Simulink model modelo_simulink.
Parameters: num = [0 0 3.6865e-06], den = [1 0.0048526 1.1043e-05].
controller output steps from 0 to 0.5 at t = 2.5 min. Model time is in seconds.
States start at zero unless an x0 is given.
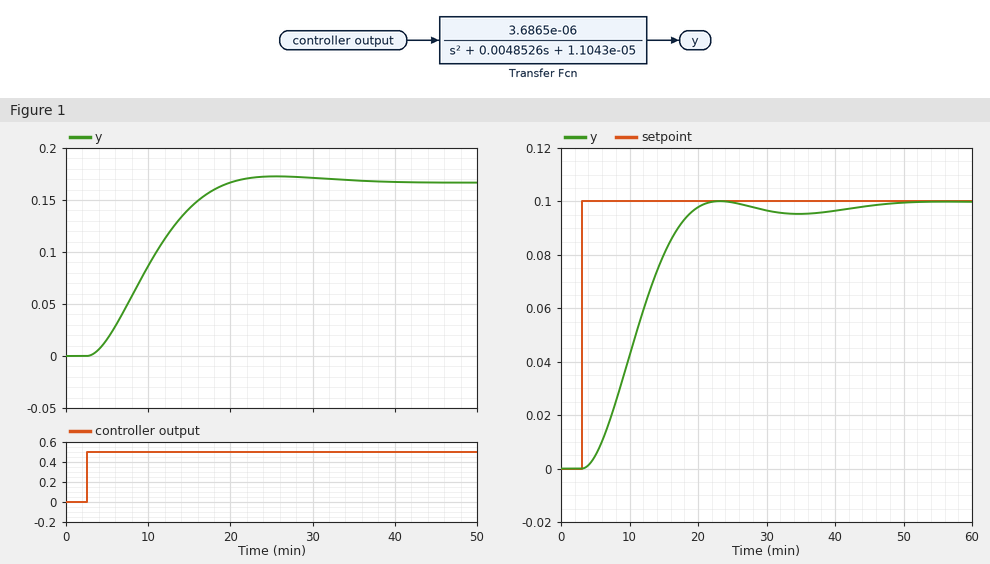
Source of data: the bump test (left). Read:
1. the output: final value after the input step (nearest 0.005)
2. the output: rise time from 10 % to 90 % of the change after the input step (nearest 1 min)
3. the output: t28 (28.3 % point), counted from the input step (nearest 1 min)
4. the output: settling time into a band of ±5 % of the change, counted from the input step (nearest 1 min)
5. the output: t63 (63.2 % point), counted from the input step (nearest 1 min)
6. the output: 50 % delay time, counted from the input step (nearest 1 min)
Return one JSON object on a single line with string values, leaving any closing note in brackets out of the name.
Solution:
{"the output: final value after the input step": "0.165", "the output: rise time from 10 % to 90 % of the change after the input step": "11 min", "the output: t28 (28.3 % point), counted from the input step": "5 min", "the output: settling time into a band of ±5 % of the change, counted from the input step": "15 min", "the output: t63 (63.2 % point), counted from the input step": "9 min", "the output: 50 % delay time, counted from the input step": "7 min"}
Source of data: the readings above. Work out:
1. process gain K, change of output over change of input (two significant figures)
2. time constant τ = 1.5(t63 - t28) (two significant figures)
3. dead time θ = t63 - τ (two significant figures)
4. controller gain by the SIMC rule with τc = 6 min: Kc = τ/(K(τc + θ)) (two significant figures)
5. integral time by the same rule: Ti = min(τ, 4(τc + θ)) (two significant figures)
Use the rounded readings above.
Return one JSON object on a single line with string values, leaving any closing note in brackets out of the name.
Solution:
{"process gain K, change of output over change of input": "0.33", "time constant τ = 1.5(t63 - t28)": "6.0 min", "dead time θ = t63 - τ": "3.0 min", "controller gain by the SIMC rule with τc = 6 min: Kc = τ/(K(τc + θ))": "2.0", "integral time by the same rule: Ti = min(τ, 4(τc + θ))": "6.0 min"}
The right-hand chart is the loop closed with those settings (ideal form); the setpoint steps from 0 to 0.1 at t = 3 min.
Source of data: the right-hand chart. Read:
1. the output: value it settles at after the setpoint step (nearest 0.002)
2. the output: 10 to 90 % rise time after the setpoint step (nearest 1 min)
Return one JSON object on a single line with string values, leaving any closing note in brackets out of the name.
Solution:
{"the output: value it settles at after the setpoint step": "0.100", "the output: 10 to 90 % rise time after the setpoint step": "11 min"}
